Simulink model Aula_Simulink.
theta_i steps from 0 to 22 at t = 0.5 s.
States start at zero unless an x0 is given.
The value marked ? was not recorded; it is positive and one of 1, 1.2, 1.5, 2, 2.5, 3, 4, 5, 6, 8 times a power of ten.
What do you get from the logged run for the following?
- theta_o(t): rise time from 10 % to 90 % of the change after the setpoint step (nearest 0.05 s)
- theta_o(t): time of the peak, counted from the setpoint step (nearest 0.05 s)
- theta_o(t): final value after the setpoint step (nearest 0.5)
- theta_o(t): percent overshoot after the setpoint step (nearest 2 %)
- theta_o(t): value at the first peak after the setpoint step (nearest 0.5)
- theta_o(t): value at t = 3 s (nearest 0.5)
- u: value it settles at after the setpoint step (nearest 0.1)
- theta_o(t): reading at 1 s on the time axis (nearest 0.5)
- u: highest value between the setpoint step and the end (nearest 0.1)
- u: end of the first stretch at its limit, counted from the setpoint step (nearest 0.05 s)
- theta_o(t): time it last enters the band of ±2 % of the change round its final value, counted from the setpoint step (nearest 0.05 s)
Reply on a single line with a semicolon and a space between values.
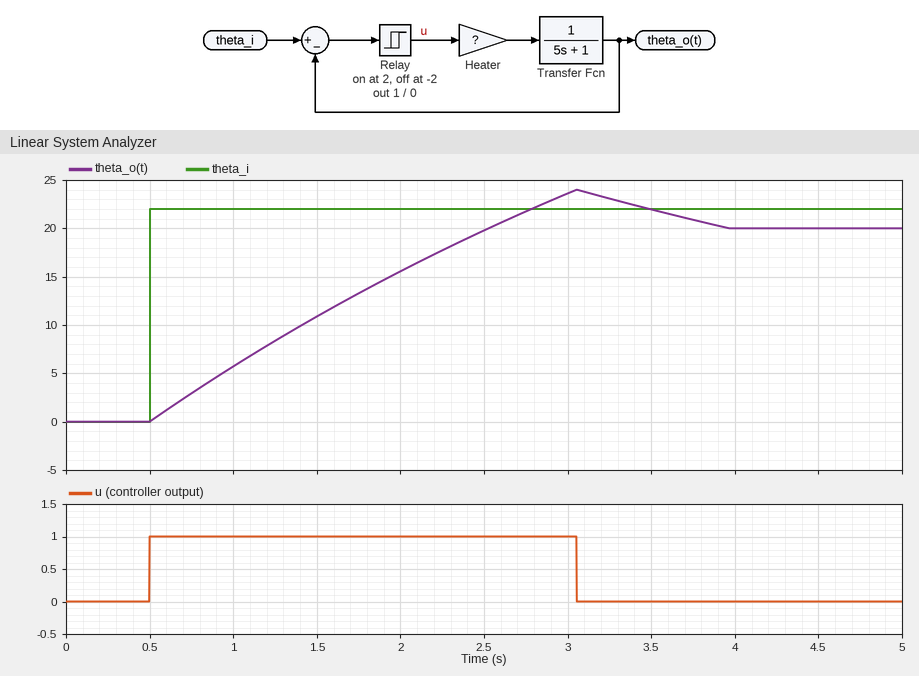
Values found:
1.60 s; 2.55 s; 20.0; 20 %; 24.0; 23.5; 0.0; 5.5; 1.0; 2.55 s; 3.35 s
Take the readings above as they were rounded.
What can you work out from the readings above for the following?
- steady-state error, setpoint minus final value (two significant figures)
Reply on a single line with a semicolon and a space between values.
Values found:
2.0
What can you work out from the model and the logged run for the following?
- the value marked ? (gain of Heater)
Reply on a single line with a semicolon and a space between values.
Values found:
60
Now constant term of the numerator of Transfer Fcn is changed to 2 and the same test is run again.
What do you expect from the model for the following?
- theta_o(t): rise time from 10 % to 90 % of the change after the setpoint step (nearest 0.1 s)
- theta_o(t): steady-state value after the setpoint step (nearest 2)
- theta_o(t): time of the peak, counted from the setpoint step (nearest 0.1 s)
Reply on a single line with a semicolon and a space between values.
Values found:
0.7 s; 20; 1.1 s
